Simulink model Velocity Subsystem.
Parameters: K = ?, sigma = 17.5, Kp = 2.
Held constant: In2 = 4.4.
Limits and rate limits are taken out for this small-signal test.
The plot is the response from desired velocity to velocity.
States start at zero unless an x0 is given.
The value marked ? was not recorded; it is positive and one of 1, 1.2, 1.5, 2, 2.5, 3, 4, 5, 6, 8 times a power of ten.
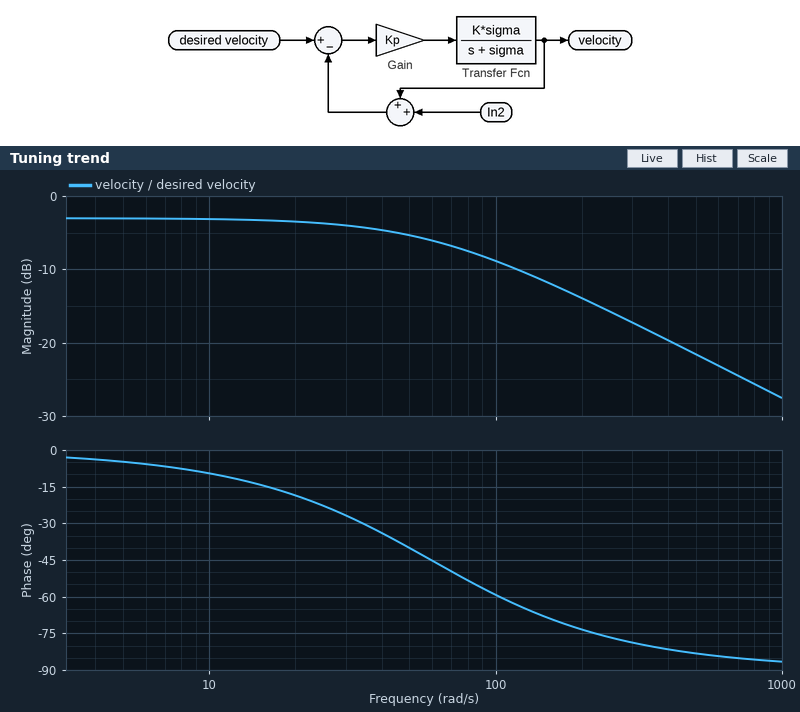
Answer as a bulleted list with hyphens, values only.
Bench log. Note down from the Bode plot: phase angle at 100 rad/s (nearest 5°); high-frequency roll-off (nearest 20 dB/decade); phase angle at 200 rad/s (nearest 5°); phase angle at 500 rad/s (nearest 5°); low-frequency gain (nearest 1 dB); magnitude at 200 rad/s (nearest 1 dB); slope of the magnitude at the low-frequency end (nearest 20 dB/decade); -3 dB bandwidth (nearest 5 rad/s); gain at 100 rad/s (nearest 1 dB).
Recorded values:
- -60°
- -20 dB/decade
- -75°
- -85°
- -3 dB
- -14 dB
- 0 dB/decade
- 60 rad/s
- -9 dB
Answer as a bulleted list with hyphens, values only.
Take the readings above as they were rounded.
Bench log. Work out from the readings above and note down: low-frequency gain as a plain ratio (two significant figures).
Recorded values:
- 0.71
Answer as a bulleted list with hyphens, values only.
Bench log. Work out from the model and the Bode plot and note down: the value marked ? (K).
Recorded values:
- 1.2
